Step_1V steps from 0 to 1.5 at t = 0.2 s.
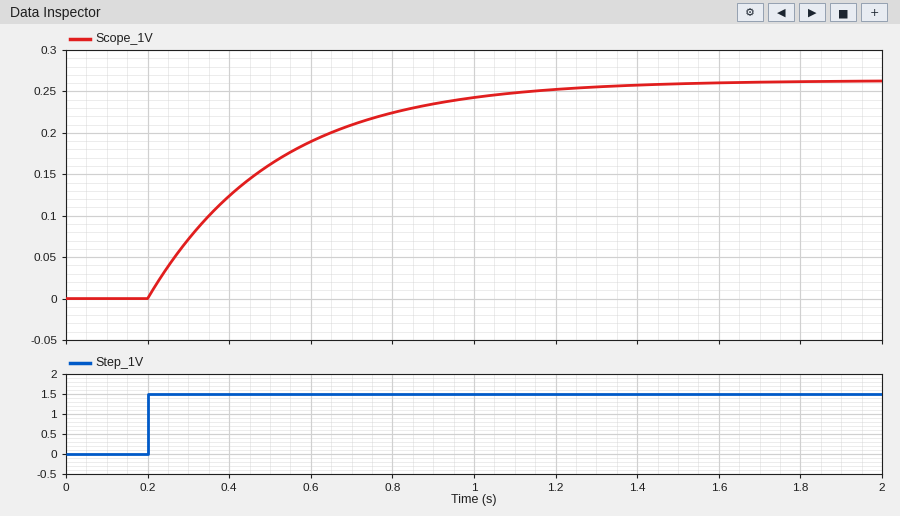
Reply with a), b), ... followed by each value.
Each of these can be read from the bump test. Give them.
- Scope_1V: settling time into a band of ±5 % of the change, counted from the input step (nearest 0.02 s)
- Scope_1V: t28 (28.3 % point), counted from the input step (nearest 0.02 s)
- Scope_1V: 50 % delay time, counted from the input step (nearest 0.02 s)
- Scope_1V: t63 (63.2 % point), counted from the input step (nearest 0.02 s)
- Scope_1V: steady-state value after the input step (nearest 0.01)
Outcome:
a) 0.94 s
b) 0.10 s
c) 0.22 s
d) 0.32 s
e) 0.26
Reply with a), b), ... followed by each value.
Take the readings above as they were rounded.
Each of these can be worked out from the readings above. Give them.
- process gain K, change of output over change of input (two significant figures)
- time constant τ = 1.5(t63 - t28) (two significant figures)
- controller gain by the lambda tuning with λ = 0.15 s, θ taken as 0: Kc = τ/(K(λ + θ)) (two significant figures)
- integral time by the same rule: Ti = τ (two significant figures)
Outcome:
a) 0.17
b) 0.33 s
c) 13
d) 0.33 s
